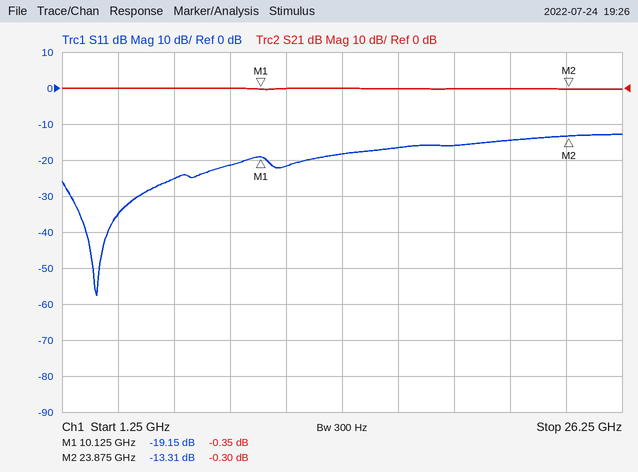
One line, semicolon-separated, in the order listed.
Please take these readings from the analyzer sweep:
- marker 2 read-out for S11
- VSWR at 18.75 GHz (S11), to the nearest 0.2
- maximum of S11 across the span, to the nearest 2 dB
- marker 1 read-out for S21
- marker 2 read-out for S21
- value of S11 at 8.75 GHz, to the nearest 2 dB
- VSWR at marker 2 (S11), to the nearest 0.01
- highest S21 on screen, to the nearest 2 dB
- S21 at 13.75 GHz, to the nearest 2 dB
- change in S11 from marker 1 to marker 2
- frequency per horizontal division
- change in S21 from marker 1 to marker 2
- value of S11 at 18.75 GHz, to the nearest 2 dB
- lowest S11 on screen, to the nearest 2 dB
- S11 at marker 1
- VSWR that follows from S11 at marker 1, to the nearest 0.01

-13.31 dB; 1.4; -12 dB; -0.35 dB; -0.30 dB; -22 dB; 1.55; 0 dB; 0 dB; 5.84 dB; 2.5 GHz; 0.05 dB; -16 dB; -58 dB; -19.15 dB; 1.25
